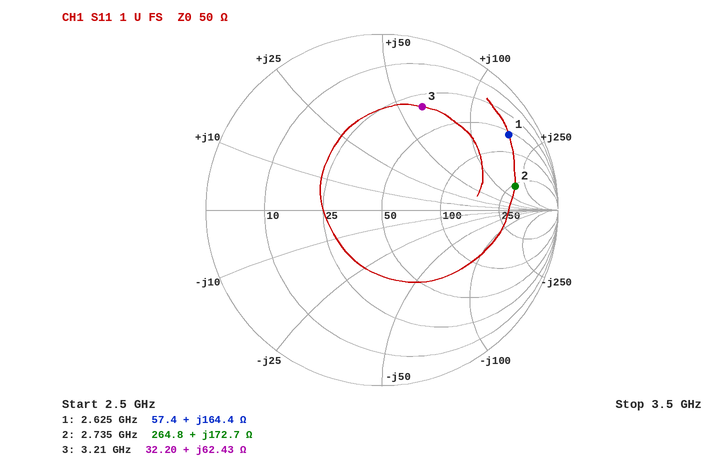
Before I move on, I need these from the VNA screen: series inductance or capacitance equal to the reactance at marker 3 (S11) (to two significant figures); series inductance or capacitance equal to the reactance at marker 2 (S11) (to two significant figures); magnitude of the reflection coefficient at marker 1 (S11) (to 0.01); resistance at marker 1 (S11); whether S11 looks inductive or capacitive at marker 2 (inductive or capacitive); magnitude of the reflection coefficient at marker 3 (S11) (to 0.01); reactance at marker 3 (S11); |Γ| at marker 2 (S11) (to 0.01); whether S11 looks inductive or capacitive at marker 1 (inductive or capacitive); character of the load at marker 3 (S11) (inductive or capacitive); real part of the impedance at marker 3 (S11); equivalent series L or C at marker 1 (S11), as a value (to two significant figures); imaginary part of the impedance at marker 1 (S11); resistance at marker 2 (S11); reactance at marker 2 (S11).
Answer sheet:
3.1 nH
10 nH
0.84
57.4 Ω
inductive
0.63
+62.43 Ω
0.77
inductive
inductive
32.20 Ω
10.0 nH
+164.4 Ω
264.8 Ω
+172.7 Ω
